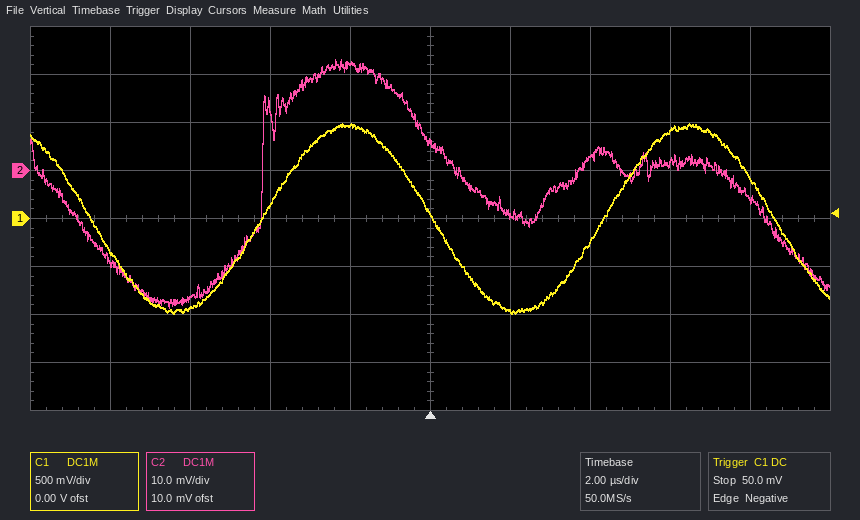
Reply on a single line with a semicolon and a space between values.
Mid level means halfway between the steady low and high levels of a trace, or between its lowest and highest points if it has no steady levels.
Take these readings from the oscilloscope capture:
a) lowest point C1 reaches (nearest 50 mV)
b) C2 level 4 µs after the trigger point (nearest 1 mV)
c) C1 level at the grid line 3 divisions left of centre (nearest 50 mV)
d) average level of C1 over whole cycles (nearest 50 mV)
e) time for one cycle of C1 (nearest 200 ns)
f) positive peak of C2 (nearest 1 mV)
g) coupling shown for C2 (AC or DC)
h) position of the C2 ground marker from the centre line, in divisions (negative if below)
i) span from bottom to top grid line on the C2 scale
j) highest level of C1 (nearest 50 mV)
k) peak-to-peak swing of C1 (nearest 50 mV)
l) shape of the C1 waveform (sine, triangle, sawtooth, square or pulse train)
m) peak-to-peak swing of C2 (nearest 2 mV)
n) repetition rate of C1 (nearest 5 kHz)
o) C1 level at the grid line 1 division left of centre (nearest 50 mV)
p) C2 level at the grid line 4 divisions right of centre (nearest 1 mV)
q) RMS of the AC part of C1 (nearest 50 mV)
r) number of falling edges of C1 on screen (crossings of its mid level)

-1.00 V; 3 mV; -950 mV; 0 mV; 8.6 µs; 23 mV; DC; +1.0 div; 80 mV; 1.00 V; 2.00 V; sine; 52 mV; 115 kHz; 950 mV; -6 mV; 700 mV; 3
